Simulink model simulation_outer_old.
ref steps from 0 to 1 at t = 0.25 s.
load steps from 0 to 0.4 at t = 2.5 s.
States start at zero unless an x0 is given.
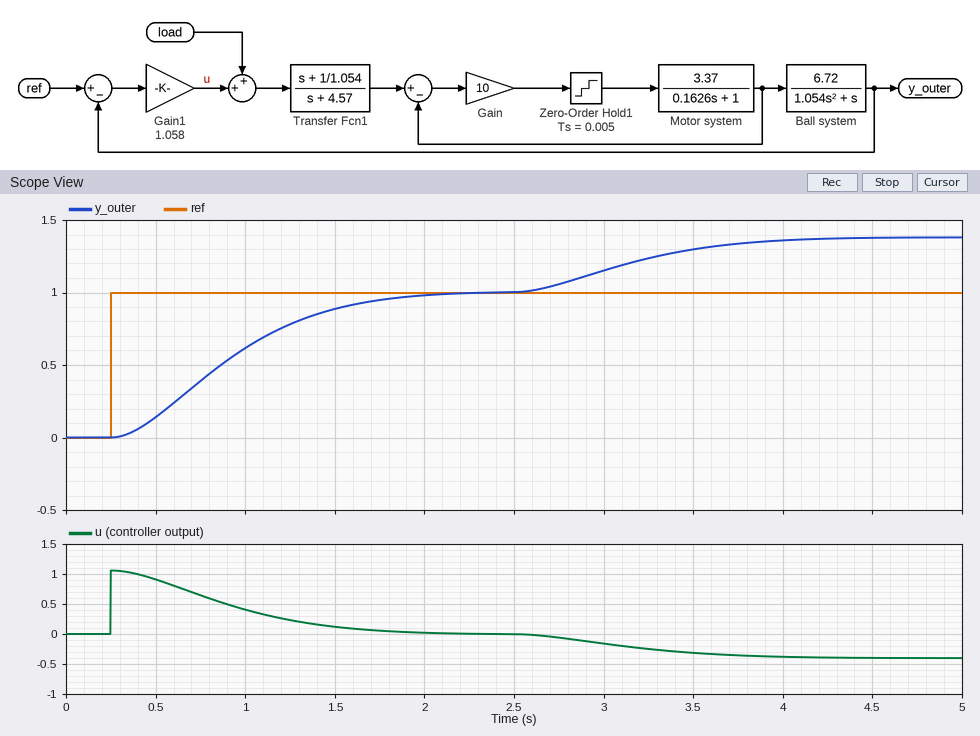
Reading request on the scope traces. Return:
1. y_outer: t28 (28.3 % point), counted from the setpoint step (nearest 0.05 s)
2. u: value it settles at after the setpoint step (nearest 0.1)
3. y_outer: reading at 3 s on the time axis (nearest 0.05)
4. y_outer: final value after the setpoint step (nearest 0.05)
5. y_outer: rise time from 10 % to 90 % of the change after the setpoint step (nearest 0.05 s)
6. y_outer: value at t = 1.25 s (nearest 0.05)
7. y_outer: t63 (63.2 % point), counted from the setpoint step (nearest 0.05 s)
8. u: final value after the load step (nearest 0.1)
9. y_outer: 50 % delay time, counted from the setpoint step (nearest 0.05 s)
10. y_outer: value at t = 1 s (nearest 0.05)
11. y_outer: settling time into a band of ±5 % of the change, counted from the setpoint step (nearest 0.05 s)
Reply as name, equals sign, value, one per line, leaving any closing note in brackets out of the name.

y_outer: t28 (28.3 % point), counted from the setpoint step = 0.40 s
u: value it settles at after the setpoint step = 0.0
y_outer: reading at 3 s on the time axis = 1.15
y_outer: final value after the setpoint step = 1.00
y_outer: rise time from 10 % to 90 % of the change after the setpoint step = 1.10 s
y_outer: value at t = 1.25 s = 0.80
y_outer: t63 (63.2 % point), counted from the setpoint step = 0.75 s
u: final value after the load step = -0.4
y_outer: 50 % delay time, counted from the setpoint step = 0.60 s
y_outer: value at t = 1 s = 0.60
y_outer: settling time into a band of ±5 % of the change, counted from the setpoint step = 1.50 s
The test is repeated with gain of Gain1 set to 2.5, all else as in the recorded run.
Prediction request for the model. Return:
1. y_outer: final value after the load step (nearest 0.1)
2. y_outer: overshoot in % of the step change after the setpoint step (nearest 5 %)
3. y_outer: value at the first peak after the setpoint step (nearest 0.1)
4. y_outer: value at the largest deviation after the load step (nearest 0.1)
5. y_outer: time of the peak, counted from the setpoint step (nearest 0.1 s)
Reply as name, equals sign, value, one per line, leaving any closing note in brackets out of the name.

y_outer: final value after the load step = 1.2
y_outer: overshoot in % of the step change after the setpoint step = 10 %
y_outer: value at the first peak after the setpoint step = 1.1
y_outer: value at the largest deviation after the load step = 1.2
y_outer: time of the peak, counted from the setpoint step = 1.0 s
